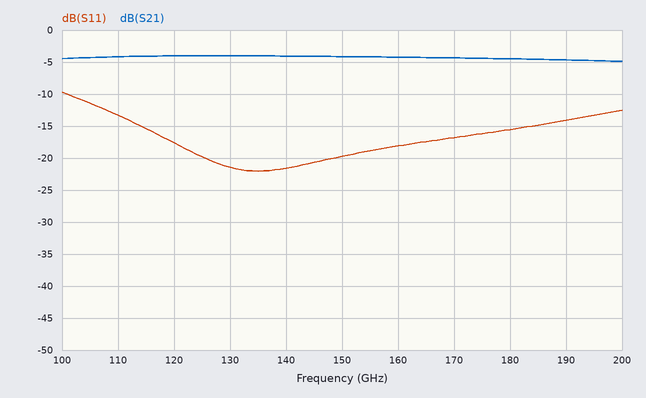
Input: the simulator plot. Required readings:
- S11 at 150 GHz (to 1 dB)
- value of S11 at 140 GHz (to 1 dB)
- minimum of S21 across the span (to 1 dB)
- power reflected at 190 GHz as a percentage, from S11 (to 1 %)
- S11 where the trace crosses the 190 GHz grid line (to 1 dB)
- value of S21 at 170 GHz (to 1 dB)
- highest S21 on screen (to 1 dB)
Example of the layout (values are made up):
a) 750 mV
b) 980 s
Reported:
a) -20 dB
b) -22 dB
c) -5 dB
d) 4 %
e) -14 dB
f) -4 dB
g) -4 dB
